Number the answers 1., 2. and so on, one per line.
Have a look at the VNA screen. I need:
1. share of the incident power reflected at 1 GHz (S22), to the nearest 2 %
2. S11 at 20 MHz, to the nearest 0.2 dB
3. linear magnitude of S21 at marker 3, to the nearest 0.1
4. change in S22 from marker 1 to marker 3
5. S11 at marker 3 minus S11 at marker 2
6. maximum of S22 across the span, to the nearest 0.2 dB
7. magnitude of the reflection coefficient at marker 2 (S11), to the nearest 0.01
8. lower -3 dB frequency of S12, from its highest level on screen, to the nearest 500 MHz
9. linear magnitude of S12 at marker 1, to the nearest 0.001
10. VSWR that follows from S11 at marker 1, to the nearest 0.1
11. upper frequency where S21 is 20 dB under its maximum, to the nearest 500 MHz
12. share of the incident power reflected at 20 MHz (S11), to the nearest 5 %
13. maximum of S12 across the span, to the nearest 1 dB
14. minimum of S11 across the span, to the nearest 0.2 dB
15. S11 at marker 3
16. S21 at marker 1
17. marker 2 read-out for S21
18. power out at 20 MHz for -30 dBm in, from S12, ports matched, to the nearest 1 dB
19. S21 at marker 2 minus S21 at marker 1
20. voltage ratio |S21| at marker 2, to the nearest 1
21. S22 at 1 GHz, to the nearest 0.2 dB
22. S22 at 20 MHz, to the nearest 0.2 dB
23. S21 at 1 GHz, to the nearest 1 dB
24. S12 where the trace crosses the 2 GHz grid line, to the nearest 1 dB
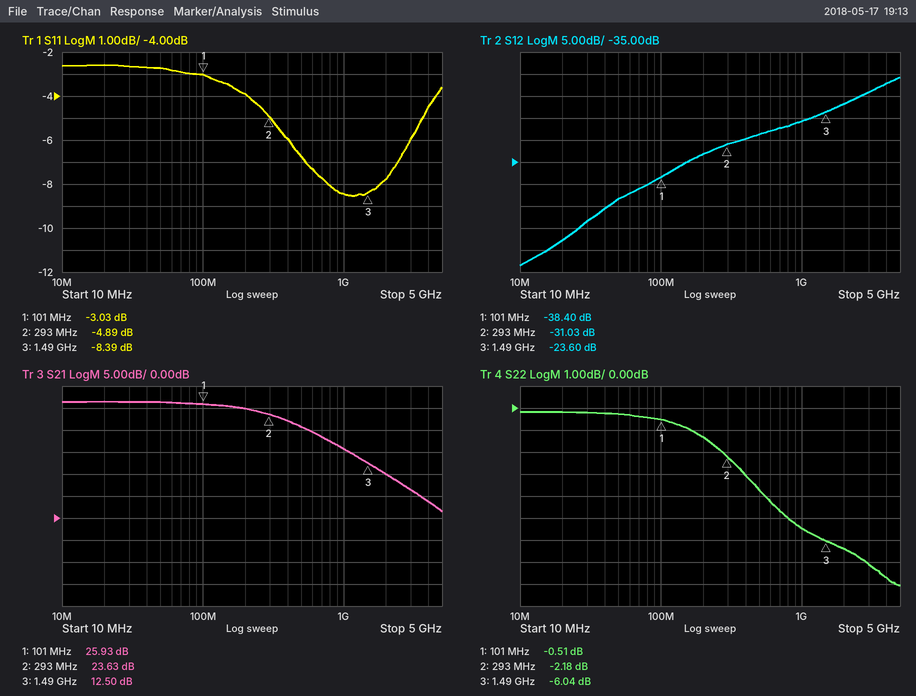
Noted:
1. 28 %
2. -2.6 dB
3. 4.2
4. -5.53 dB
5. -3.50 dB
6. -0.2 dB
7. 0.57
8. 3.0 GHz
9. 0.012
10. 5.8
11. 3.0 GHz
12. 55 %
13. -16 dB
14. -8.6 dB
15. -8.39 dB
16. 25.93 dB
17. 23.63 dB
18. -83 dBm
19. -2.30 dB
20. 15
21. -5.4 dB
22. -0.2 dB
23. 16 dB
24. -22 dB
